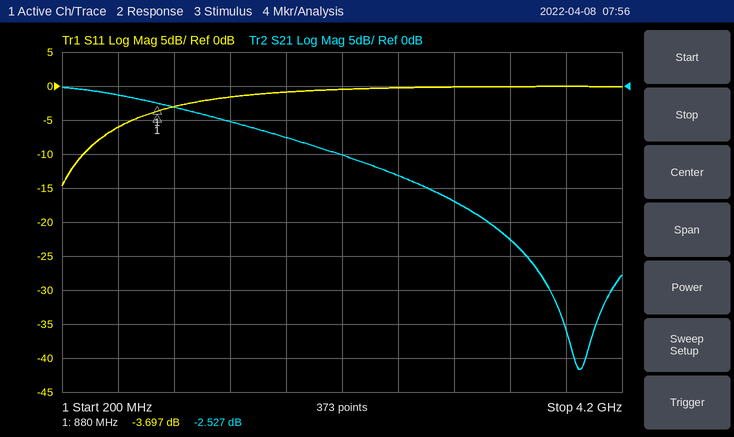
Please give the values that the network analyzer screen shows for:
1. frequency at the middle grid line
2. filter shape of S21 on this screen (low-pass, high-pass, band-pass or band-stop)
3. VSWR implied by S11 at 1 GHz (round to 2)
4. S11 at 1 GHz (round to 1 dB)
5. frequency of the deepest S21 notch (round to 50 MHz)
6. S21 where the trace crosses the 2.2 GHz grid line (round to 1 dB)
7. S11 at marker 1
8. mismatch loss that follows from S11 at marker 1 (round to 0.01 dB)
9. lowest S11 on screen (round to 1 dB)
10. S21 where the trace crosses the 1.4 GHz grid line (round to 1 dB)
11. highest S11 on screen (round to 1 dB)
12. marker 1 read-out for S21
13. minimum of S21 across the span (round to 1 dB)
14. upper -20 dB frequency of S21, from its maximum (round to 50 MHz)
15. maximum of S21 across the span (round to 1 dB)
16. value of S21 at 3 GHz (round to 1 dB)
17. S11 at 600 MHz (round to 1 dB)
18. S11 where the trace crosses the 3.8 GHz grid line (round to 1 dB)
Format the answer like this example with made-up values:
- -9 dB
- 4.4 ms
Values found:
- 2.2 GHz
- low-pass
- 6
- -3 dB
- 3.90 GHz
- -10 dB
- -3.697 dB
- 2.42 dB
- -15 dB
- -5 dB
- 0 dB
- -2.527 dB
- -42 dB
- 3.25 GHz
- 0 dB
- -17 dB
- -6 dB
- 0 dB
